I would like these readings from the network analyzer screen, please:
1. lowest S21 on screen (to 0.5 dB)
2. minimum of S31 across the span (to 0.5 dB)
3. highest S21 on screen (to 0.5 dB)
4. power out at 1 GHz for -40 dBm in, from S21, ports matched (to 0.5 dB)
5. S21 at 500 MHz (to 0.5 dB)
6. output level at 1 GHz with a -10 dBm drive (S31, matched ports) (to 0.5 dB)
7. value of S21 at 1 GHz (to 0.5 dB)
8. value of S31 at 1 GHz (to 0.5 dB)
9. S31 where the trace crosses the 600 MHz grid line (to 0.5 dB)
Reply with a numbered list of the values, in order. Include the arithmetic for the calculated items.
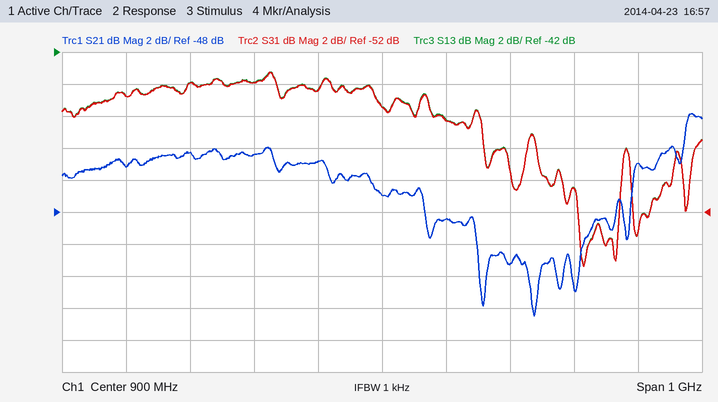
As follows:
1. -54.5 dB
2. -55.5 dB
3. -42.0 dB
4. -40 dBm + (-48.5 dB) = -88.5 dBm
5. -45.0 dB
6. -10 dBm + (-46.5 dB) = -56.5 dBm
7. -48.5 dB
8. -46.5 dB
9. -44.0 dB
